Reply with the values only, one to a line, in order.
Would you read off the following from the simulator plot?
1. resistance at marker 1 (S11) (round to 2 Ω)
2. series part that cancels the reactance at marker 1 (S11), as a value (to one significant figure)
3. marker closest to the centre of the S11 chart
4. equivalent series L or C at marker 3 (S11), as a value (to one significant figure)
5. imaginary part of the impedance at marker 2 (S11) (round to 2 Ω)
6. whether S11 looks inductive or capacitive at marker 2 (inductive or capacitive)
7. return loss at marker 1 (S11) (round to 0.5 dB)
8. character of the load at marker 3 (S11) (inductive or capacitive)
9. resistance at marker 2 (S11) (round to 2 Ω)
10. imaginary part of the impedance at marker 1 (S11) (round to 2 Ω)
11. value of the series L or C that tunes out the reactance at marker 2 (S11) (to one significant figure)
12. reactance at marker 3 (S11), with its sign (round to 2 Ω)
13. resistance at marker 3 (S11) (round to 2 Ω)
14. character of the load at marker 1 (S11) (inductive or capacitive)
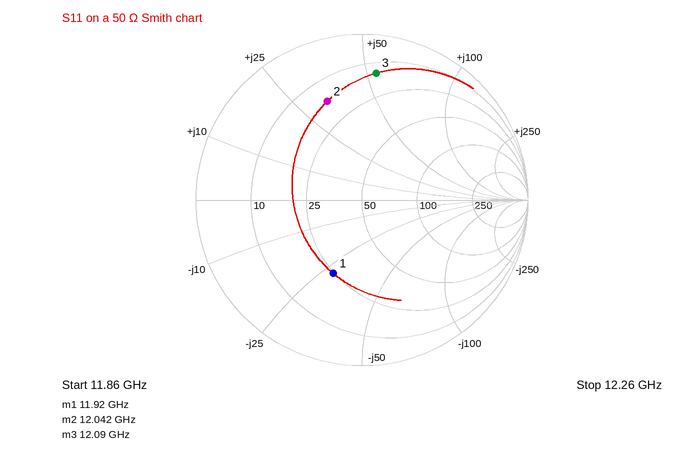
24 Ω
400 pH
marker 1
700 pH
+32 Ω
inductive
6.5 dB
inductive
16 Ω
-28 Ω
400 fF
+54 Ω
14 Ω
capacitive
